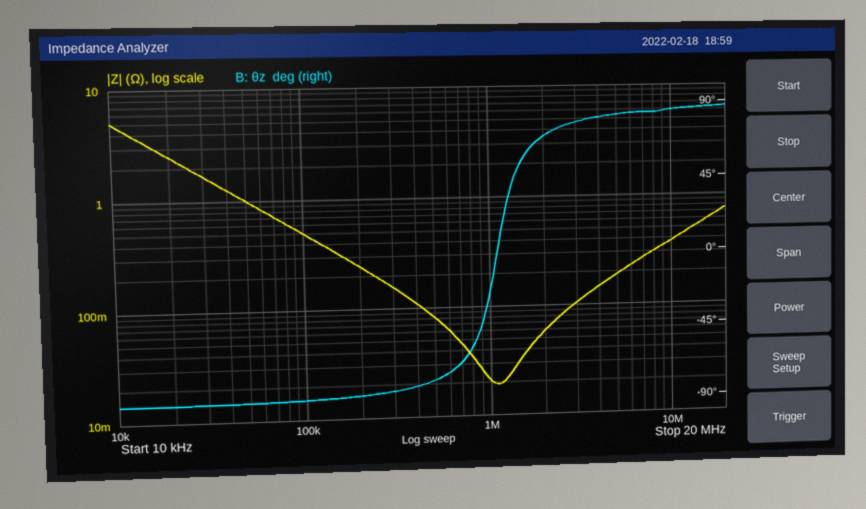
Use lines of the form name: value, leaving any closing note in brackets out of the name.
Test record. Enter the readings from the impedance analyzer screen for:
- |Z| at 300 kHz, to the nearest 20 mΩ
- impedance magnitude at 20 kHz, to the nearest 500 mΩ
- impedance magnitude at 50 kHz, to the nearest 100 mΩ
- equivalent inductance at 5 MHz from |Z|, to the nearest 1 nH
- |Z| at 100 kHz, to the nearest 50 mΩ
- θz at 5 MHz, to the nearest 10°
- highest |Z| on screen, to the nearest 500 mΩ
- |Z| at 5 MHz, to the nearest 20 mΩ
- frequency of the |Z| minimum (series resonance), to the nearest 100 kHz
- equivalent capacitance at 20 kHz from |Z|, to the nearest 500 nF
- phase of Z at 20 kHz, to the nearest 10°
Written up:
|Z| at 300 kHz, to the nearest 20 mΩ: 160 mΩ
impedance magnitude at 20 kHz, to the nearest 500 mΩ: 2.5 Ω
impedance magnitude at 50 kHz, to the nearest 100 mΩ: 1.0 Ω
equivalent inductance at 5 MHz from |Z|, to the nearest 1 nH: 6 nH
|Z| at 100 kHz, to the nearest 50 mΩ: 500 mΩ
θz at 5 MHz, to the nearest 10°: 80°
highest |Z| on screen, to the nearest 500 mΩ: 5.0 Ω
|Z| at 5 MHz, to the nearest 20 mΩ: 180 mΩ
frequency of the |Z| minimum (series resonance), to the nearest 100 kHz: 1.1 MHz
equivalent capacitance at 20 kHz from |Z|, to the nearest 500 nF: 3.0 µF
phase of Z at 20 kHz, to the nearest 10°: -90°
